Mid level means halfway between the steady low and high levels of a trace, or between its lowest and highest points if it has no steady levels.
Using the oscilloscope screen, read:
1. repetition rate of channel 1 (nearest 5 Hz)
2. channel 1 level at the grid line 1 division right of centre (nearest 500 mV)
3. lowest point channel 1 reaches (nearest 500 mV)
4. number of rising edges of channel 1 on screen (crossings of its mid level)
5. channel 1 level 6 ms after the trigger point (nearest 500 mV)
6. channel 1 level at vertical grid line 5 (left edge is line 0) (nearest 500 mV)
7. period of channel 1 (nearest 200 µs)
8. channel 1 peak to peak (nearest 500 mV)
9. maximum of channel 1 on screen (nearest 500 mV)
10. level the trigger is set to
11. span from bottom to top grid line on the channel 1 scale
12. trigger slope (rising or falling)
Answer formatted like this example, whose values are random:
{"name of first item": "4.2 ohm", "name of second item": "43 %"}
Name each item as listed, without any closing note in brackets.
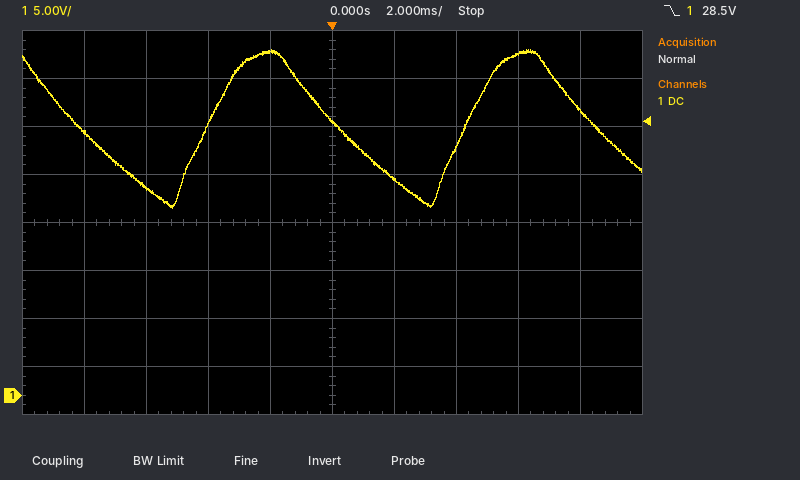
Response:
{"repetition rate of channel 1": "120 Hz", "channel 1 level at the grid line 1 division right of centre": "22.5 V", "lowest point channel 1 reaches": "19.5 V", "number of rising edges of channel 1 on screen": "2", "channel 1 level 6 ms after the trigger point": "35.5 V", "channel 1 level at vertical grid line 5 (left edge is line 0)": "28.5 V", "period of channel 1": "8.4 ms", "channel 1 peak to peak": "16.5 V", "maximum of channel 1 on screen": "36.0 V", "level the trigger is set to": "28.5 V", "span from bottom to top grid line on the channel 1 scale": "40 V", "trigger slope": "falling"}
